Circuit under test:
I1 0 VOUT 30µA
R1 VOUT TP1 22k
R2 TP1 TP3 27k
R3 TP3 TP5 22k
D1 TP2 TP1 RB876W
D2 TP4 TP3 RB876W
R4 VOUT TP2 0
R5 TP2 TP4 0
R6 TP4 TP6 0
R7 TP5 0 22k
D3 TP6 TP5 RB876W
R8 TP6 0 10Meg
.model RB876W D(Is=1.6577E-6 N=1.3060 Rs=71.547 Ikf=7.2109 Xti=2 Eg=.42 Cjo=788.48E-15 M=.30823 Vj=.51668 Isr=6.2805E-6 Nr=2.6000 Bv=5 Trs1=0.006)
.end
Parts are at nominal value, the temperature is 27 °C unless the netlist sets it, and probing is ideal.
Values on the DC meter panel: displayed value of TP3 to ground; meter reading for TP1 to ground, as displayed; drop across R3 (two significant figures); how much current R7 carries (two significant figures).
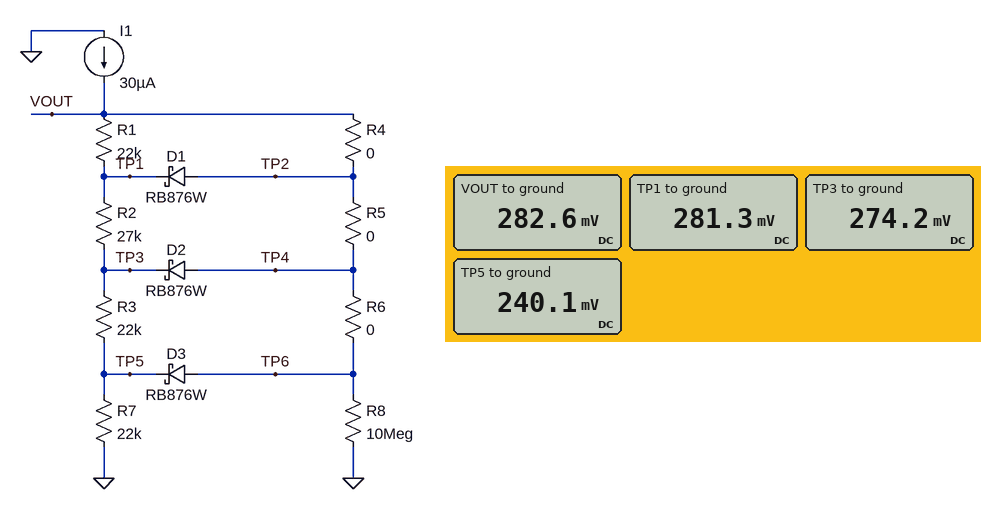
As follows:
274.2 mV
281.3 mV
34 mV
11 µA
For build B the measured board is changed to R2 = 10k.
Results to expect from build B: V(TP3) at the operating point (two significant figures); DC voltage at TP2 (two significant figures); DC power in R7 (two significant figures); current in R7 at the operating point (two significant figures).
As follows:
420 mV
430 mV
6.2 µW
17 µA
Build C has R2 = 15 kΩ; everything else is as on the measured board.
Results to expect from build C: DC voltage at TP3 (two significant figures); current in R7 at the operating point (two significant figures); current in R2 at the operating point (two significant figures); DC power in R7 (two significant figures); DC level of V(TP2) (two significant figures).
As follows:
330 mV
13 µA
440 nA
3.9 µW
340 mV
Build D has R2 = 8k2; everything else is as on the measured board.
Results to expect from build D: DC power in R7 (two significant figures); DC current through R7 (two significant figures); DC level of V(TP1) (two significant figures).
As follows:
8.5 µW
20 µA
490 mV
